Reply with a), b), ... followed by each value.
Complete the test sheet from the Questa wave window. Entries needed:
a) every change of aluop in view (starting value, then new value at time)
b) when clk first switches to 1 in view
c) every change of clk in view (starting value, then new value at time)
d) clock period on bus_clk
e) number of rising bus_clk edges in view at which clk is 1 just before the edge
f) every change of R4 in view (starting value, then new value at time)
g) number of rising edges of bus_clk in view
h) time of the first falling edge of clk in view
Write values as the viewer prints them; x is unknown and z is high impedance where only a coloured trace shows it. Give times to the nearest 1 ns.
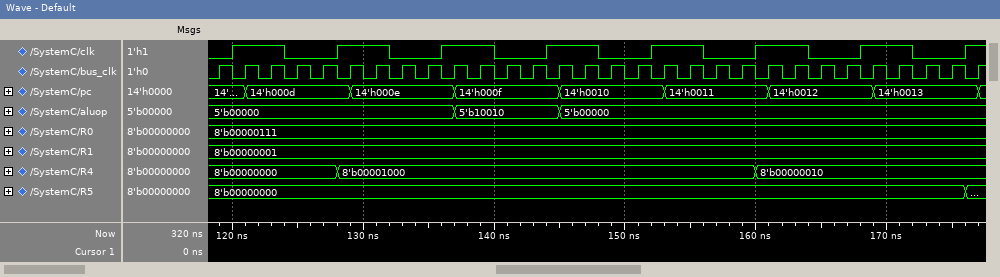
a) 5'b00000, 5'b10010 at 137 ns, 5'b00000 at 145 ns
b) 120 ns
c) 0, 1 at 120 ns, 0 at 124 ns, 1 at 128 ns, 0 at 132 ns, 1 at 136 ns, 0 at 140 ns, 1 at 144 ns, 0 at 148 ns, 1 at 152 ns, 0 at 156 ns, 1 at 160 ns, 0 at 164 ns, 1 at 168 ns, 0 at 172 ns, 1 at 176 ns
d) 2 ns
e) 15
f) 8'b00000000, 8'b00001000 at 128 ns, 8'b00000010 at 160 ns
g) 30
h) 124 ns
